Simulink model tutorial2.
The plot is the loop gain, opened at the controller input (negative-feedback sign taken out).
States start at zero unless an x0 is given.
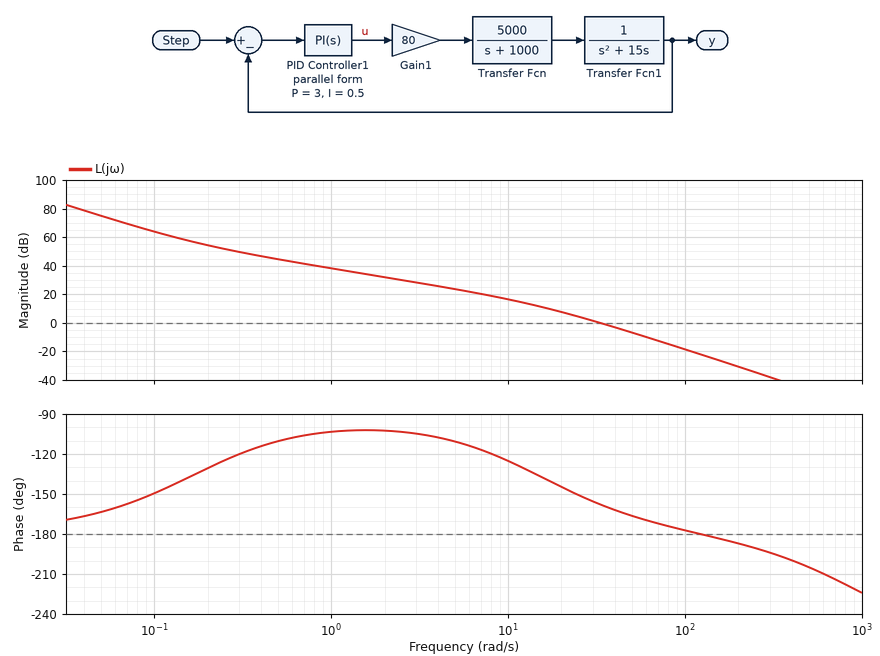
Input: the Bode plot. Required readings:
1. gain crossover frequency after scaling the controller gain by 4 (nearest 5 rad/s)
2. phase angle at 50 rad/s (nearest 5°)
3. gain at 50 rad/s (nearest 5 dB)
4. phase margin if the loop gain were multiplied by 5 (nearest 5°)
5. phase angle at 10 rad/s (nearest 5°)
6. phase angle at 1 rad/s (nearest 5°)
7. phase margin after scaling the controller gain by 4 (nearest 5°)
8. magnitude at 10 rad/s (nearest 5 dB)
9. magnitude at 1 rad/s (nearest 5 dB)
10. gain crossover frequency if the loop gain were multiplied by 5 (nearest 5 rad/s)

70 rad/s
-165°
-5 dB
5°
-125°
-105°
10°
15 dB
40 dB
75 rad/s
